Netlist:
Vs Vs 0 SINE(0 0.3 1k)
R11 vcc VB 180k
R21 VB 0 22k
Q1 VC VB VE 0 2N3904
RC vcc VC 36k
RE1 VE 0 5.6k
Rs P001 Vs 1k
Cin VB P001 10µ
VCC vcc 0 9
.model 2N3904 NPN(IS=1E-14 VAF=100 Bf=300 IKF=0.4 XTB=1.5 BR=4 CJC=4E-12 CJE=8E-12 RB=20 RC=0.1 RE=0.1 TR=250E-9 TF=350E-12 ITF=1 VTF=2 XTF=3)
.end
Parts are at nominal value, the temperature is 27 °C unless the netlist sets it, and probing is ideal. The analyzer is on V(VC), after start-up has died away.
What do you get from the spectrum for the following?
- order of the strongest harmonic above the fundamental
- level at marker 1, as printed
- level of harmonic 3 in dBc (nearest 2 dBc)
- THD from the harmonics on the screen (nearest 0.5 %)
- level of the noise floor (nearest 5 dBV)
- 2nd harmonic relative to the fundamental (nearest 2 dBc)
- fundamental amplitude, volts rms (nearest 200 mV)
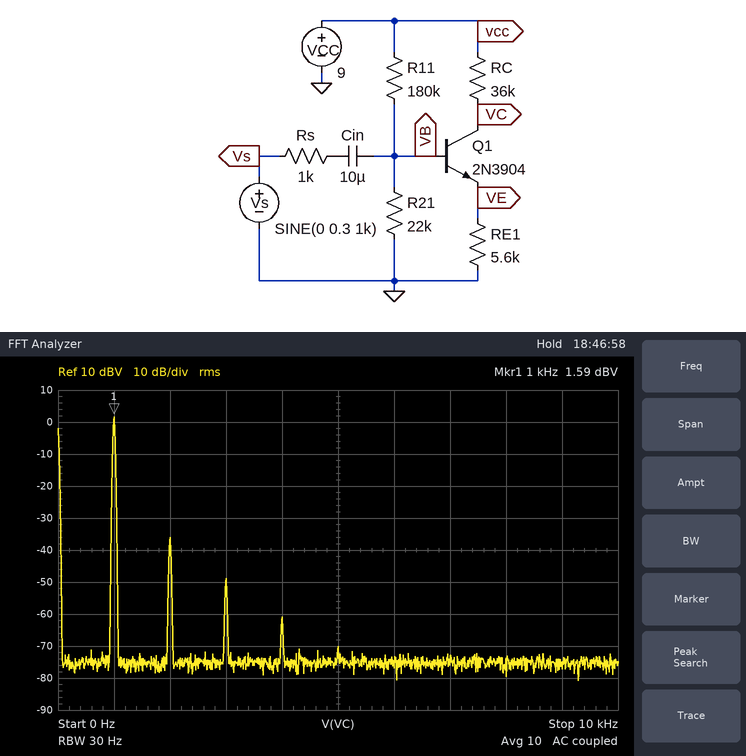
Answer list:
2
1.59 dBV
-50 dBc
1.5 %
-75 dBV
-38 dBc
1.2 V
